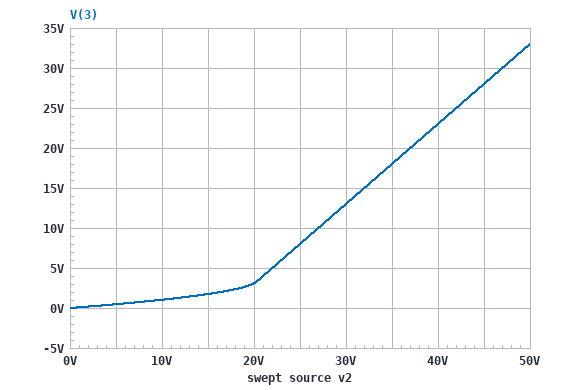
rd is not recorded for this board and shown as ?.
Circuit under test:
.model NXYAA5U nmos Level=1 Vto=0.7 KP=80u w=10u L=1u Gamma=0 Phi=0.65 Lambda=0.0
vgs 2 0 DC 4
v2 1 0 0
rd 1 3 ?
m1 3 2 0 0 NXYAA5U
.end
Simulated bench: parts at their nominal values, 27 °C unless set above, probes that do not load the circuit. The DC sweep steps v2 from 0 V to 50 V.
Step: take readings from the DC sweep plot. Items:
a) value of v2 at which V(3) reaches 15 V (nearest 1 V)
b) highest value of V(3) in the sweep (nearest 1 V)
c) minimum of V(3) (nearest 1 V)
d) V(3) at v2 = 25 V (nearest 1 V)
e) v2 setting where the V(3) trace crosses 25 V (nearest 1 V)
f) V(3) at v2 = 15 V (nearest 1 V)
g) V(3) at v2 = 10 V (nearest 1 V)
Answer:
32 V
33 V
0 V
8 V
42 V
2 V
1 V
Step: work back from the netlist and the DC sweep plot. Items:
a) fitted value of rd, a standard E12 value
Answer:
3.9 kΩ
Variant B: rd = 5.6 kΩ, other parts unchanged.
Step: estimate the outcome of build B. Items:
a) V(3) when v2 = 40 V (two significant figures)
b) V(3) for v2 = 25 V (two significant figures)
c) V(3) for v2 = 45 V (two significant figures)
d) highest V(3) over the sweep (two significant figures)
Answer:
16 V
2.4 V
21 V
26 V
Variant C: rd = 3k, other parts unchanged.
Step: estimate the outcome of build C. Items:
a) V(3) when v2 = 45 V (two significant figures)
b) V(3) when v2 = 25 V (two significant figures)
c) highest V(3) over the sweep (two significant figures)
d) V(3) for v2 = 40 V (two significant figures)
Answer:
32 V
12 V
37 V
27 V
